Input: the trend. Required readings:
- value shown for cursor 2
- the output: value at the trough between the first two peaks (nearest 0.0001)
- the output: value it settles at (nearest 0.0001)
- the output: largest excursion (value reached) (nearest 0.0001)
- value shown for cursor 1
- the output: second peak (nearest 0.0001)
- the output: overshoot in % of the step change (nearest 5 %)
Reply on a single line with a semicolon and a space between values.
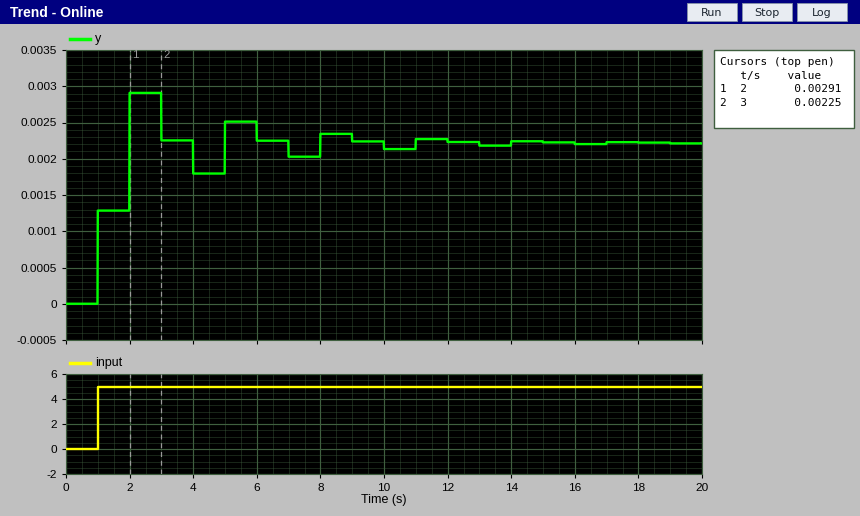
0.00225; 0.0018; 0.0022; 0.0029; 0.00291; 0.0025; 30 %
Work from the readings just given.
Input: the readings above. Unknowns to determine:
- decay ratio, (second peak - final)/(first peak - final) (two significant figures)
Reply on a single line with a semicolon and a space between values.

0.43
